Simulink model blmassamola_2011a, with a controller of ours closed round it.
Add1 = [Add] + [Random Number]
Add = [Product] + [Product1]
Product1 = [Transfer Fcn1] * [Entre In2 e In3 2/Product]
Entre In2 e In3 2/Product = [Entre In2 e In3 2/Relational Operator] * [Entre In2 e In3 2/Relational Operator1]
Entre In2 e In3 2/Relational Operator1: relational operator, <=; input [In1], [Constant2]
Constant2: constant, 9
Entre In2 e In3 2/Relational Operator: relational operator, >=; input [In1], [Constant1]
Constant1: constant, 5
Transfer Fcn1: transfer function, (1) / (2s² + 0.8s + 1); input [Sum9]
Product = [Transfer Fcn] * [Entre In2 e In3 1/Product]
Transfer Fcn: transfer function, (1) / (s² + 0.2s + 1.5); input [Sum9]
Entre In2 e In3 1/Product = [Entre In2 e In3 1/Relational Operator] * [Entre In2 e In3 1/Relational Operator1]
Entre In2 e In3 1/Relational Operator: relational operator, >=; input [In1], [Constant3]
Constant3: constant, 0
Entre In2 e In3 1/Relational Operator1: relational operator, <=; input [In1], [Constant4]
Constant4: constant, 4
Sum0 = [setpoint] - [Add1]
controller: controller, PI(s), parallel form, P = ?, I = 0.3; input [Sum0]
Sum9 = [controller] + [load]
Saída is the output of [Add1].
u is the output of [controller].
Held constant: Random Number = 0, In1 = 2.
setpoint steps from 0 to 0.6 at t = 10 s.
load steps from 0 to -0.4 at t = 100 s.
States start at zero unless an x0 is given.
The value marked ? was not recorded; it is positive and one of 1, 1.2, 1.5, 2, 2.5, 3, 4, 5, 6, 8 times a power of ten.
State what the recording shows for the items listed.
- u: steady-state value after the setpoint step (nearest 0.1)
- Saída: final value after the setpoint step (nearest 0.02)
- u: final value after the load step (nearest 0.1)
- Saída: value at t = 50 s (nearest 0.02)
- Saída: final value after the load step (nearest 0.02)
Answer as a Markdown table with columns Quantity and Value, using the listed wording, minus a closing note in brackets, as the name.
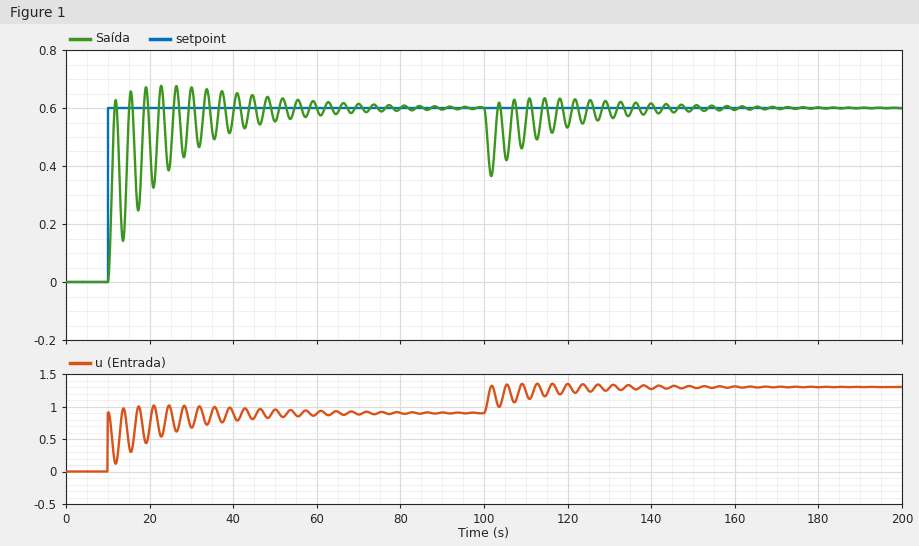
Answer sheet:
| Quantity | Value |
|---|---|
| u: steady-state value after the setpoint step | 0.9 |
| Saída: final value after the setpoint step | 0.60 |
| u: final value after the load step | 1.3 |
| Saída: value at t = 50 s | 0.56 |
| Saída: final value after the load step | 0.60 |
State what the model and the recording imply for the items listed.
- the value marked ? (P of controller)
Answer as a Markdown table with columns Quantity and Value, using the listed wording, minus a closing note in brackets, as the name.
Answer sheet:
| Quantity | Value |
|---|---|
| the value marked ? | 1.5 |
